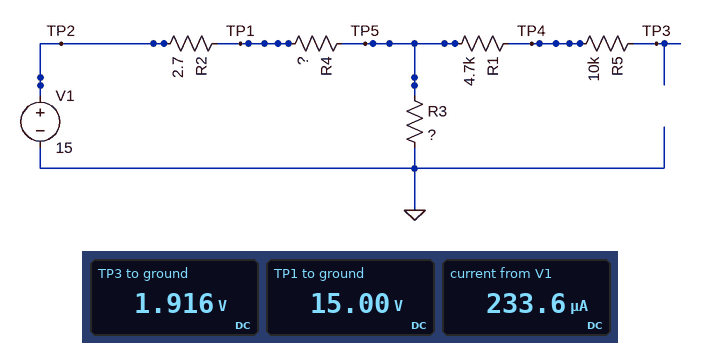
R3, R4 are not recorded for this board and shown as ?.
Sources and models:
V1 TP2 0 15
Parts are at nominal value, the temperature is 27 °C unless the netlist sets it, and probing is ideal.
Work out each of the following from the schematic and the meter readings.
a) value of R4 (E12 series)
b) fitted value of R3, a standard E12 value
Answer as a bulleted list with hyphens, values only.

- 56 kΩ
- 8.2 kΩ
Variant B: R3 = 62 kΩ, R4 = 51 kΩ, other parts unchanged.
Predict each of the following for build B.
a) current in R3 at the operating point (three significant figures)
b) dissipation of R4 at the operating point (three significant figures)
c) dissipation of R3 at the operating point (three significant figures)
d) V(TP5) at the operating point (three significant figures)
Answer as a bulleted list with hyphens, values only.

- 133 µA
- 899 µW
- 1.09 mW
- 8.23 V
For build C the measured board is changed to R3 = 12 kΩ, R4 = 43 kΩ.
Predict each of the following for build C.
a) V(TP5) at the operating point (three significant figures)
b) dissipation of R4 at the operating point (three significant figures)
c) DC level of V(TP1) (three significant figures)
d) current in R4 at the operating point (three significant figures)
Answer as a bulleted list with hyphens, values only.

- 3.27 V
- 3.20 mW
- 15.0 V
- 273 µA
